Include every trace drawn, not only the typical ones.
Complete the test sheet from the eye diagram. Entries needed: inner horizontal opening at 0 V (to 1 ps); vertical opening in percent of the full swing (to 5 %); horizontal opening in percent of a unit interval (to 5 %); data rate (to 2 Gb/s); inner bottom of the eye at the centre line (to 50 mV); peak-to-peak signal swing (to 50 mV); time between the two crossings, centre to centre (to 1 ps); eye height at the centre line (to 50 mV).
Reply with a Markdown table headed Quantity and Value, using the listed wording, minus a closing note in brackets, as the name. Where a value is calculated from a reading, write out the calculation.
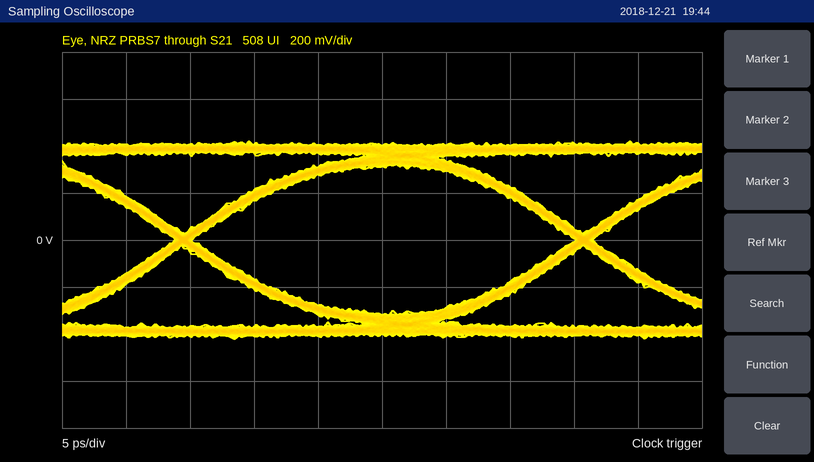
| Quantity | Value |
|---|---|
| inner horizontal opening at 0 V | 30 ps |
| vertical opening in percent of the full swing | 650 mV / 850 mV ≈ 76.5 %, so 75 % to the nearest 5 % |
| horizontal opening in percent of a unit interval | 30 ps / 31 ps ≈ 96.8 %, so 95 % to the nearest 5 % |
| data rate | 32 Gb/s |
| inner bottom of the eye at the centre line | -300 mV |
| peak-to-peak signal swing | 850 mV |
| time between the two crossings, centre to centre | 31 ps |
| eye height at the centre line | 650 mV |
